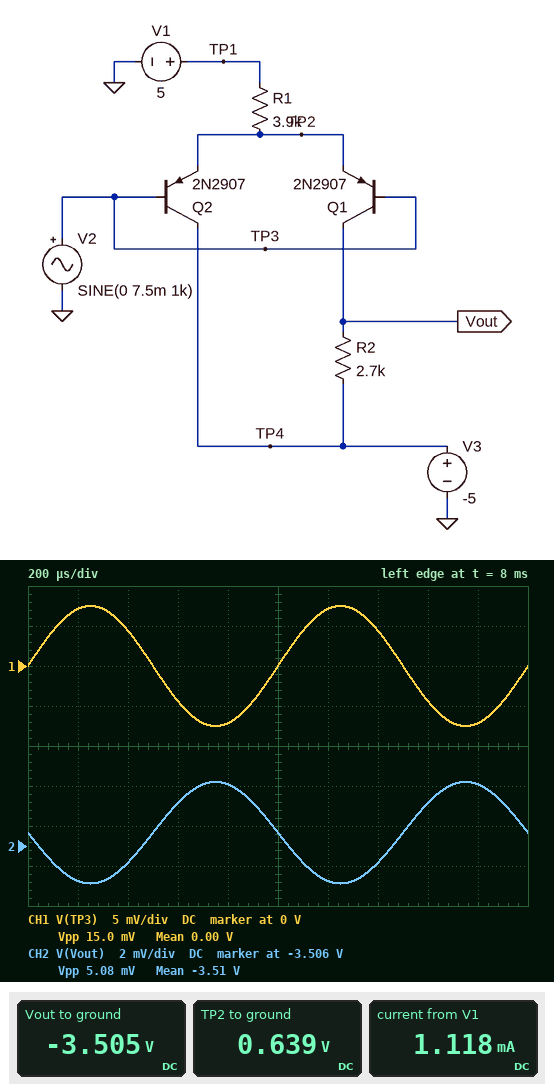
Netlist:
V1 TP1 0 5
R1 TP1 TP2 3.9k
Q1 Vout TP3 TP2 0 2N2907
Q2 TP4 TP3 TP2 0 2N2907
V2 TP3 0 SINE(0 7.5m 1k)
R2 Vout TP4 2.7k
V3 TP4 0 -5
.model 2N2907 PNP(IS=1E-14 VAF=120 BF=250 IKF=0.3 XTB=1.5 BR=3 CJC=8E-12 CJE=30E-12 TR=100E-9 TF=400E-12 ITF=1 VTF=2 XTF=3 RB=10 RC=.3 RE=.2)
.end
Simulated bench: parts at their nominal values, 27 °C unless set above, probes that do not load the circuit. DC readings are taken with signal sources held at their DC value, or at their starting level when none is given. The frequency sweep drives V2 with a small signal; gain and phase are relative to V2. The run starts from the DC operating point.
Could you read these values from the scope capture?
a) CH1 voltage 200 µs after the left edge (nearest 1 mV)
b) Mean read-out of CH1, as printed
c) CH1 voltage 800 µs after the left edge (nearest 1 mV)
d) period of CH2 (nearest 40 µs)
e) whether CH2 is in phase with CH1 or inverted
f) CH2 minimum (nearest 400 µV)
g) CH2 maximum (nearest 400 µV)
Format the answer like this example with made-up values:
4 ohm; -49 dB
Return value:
7 mV; 0.00 V; -7 mV; 1.00 ms; inverted; -3.5080 V; -3.5028 V
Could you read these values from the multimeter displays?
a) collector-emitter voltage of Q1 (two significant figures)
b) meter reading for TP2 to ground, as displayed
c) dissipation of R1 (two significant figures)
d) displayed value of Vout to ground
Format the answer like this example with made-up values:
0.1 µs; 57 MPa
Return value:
-4.1 V; 0.639 V; 4.9 mW; -3.505 V
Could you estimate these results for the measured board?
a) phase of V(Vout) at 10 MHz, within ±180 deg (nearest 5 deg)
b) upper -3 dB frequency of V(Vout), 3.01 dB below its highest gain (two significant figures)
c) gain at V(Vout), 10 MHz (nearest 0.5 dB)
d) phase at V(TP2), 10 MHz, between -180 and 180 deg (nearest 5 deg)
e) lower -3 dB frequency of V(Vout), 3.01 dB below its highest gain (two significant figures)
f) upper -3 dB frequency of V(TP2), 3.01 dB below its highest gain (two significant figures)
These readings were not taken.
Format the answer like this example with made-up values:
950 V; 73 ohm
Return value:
70 deg; 7.9 GHz; -3.5 dB; 0 deg; 11 MHz; 7.5 GHz
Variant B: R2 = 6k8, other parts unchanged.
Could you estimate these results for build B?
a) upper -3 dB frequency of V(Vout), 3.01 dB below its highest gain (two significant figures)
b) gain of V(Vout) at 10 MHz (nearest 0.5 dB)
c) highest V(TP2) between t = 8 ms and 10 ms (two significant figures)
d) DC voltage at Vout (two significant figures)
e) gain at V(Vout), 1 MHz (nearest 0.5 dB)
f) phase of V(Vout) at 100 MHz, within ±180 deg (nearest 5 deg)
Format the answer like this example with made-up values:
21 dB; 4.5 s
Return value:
7.8 GHz; -0.5 dB; 650 mV; -1.3 V; -1.5 dB; 5 deg
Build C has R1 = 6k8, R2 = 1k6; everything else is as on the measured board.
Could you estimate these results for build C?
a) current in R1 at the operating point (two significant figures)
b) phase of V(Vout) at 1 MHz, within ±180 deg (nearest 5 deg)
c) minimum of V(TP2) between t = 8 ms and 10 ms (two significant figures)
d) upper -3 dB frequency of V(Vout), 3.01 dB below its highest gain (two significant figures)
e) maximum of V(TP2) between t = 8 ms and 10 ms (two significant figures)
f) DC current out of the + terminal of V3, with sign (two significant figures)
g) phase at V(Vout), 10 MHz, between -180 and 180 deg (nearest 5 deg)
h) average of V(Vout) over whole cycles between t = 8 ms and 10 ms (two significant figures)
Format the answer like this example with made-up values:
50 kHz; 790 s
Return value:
640 µA; 155 deg; 620 mV; 7.9 GHz; 630 mV; -640 µA; 80 deg; -4.5 V
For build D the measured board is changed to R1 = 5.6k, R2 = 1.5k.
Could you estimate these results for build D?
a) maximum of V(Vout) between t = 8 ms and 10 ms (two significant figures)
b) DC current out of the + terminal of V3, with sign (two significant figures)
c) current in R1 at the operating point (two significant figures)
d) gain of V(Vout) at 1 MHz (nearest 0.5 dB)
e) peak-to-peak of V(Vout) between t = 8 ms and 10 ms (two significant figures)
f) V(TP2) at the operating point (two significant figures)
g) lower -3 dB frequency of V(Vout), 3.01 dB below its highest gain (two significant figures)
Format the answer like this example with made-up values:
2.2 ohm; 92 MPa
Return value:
-4.4 V; -780 µA; 780 µA; -17.0 dB; 2.0 mV; 630 mV; 25 MHz
